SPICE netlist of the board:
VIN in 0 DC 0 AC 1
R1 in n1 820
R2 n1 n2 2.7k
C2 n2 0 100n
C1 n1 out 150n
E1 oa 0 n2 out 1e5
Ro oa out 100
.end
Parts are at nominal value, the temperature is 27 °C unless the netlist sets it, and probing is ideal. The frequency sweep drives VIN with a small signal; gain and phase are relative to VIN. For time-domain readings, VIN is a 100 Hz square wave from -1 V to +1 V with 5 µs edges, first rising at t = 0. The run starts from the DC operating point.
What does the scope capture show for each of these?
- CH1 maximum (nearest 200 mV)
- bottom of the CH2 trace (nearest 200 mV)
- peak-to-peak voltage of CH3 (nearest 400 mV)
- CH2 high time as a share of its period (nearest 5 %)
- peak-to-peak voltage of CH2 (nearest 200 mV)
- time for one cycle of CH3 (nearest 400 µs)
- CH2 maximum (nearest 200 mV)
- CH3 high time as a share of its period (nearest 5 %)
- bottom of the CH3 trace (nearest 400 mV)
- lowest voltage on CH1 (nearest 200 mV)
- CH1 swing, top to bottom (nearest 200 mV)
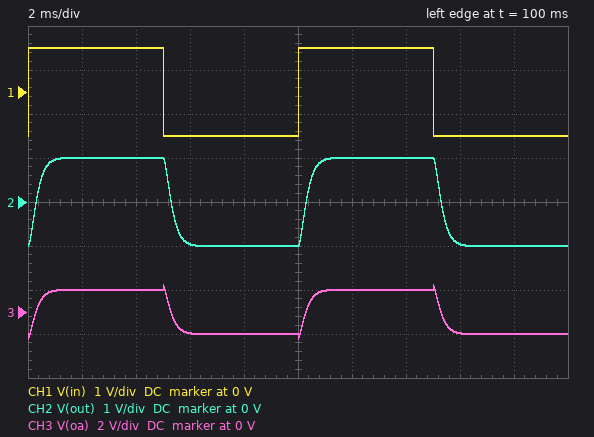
1.0 V
-1.0 V
2.4 V
50 %
2.0 V
10.0 ms
1.0 V
50 %
-1.2 V
-1.0 V
2.0 V
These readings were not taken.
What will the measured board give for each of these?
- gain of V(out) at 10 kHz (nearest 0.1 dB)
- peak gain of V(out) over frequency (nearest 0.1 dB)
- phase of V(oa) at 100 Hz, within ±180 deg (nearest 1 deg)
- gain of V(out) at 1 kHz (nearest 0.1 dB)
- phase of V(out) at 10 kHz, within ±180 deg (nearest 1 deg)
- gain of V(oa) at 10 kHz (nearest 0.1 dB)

-42.4 dB
0 dB
-13 deg
-7.0 dB
-170 deg
-17.8 dB
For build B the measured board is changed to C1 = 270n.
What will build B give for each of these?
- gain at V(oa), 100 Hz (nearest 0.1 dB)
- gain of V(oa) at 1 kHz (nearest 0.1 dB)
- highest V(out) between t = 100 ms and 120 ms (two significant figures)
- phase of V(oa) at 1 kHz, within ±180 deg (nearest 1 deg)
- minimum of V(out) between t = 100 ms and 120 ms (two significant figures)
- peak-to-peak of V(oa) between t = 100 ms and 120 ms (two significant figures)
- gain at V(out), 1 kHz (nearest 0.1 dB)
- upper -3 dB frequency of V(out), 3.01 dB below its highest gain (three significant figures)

0 dB
-6.1 dB
1.1 V
-122 deg
-1.1 V
2.5 V
-8.3 dB
639 Hz
